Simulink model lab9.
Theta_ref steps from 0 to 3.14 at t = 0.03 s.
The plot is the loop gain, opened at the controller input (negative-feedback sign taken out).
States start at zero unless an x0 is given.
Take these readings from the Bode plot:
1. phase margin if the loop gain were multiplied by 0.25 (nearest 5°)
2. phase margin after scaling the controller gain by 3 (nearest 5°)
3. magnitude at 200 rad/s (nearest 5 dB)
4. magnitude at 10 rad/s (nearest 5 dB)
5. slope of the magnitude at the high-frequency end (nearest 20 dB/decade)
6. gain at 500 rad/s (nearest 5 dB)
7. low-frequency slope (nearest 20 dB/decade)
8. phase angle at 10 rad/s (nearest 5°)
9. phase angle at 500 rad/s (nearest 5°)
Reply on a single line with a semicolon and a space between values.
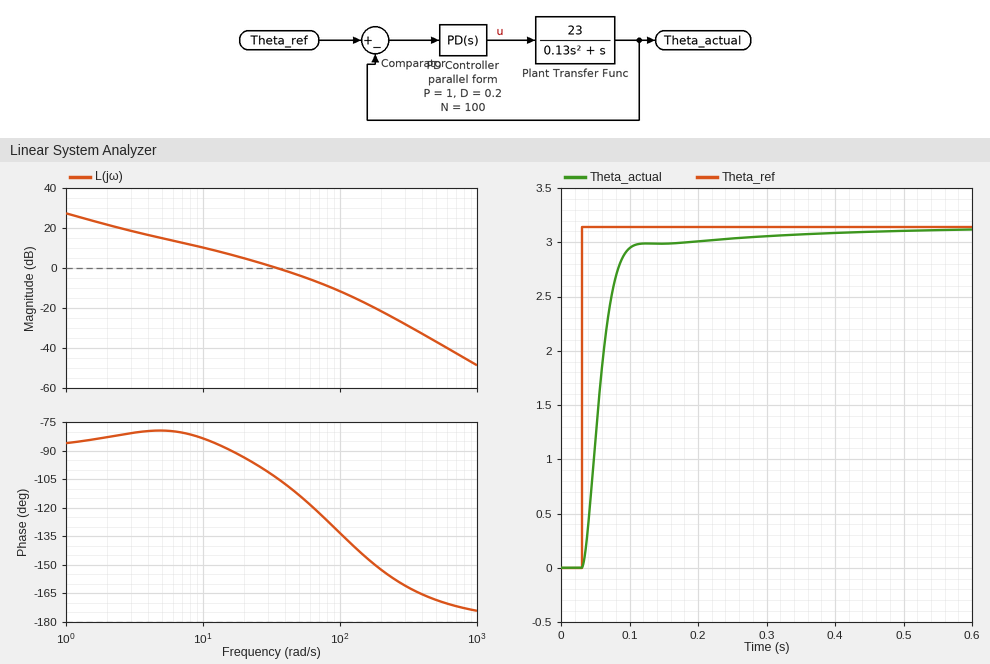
100°; 50°; -20 dB; 10 dB; -40 dB/decade; -35 dB; -20 dB/decade; -85°; -170°
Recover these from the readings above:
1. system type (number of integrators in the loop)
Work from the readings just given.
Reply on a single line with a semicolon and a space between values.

1
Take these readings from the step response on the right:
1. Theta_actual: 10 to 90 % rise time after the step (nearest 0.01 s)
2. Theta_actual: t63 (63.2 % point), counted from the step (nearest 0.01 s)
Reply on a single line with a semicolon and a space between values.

0.05 s; 0.03 s
